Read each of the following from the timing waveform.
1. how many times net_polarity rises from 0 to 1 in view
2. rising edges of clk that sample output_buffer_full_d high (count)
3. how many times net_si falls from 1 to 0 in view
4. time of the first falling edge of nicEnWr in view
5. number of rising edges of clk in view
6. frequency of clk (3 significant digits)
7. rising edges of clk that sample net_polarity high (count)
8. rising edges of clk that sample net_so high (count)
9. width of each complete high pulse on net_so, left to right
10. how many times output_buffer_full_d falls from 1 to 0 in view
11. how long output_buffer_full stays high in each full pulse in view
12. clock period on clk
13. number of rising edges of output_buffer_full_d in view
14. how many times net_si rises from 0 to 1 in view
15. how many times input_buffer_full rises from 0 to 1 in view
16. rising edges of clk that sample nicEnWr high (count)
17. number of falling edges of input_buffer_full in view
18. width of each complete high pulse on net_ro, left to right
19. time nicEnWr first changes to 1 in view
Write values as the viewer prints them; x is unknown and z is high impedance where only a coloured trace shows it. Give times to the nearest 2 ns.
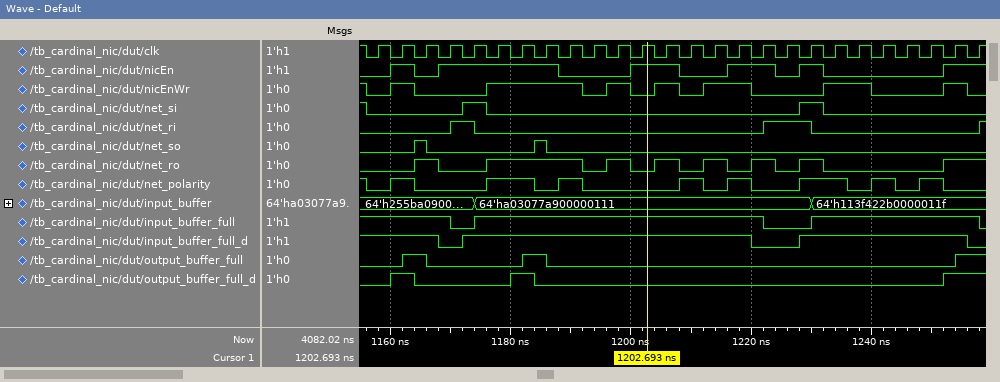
8
4
3
1156 ns
26
250 MHz
10
2
2 ns, 2 ns
2
4 ns, 4 ns
4 ns
3
2
2
12
3
4 ns, 16 ns, 4 ns, 4 ns, 4 ns, 4 ns, 4 ns
1160 ns
